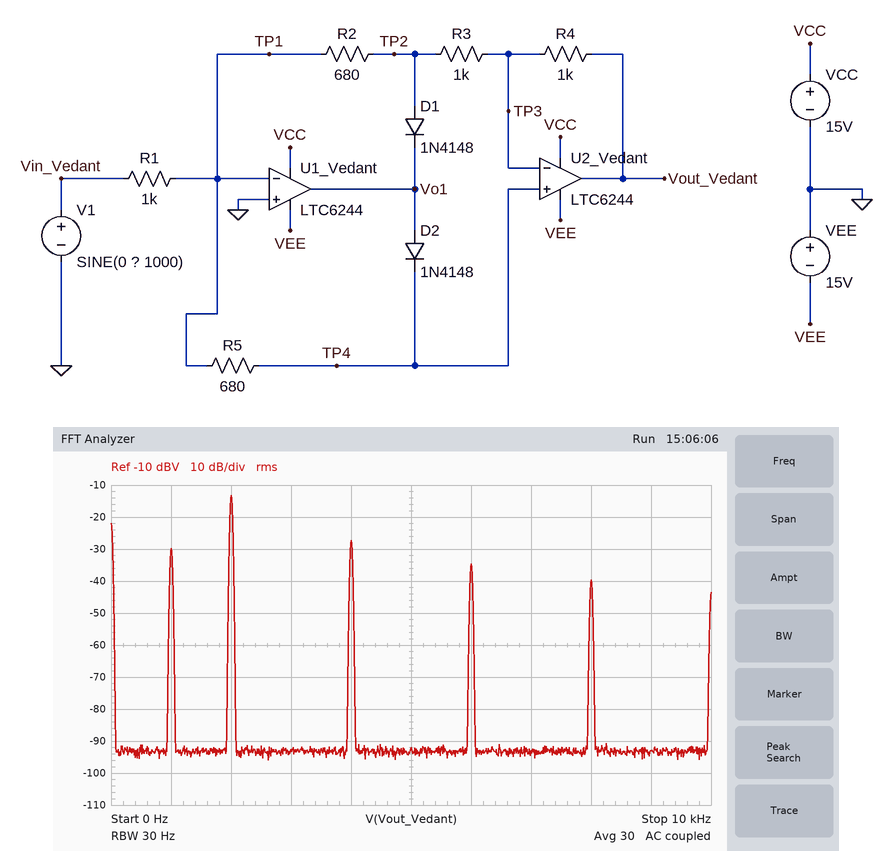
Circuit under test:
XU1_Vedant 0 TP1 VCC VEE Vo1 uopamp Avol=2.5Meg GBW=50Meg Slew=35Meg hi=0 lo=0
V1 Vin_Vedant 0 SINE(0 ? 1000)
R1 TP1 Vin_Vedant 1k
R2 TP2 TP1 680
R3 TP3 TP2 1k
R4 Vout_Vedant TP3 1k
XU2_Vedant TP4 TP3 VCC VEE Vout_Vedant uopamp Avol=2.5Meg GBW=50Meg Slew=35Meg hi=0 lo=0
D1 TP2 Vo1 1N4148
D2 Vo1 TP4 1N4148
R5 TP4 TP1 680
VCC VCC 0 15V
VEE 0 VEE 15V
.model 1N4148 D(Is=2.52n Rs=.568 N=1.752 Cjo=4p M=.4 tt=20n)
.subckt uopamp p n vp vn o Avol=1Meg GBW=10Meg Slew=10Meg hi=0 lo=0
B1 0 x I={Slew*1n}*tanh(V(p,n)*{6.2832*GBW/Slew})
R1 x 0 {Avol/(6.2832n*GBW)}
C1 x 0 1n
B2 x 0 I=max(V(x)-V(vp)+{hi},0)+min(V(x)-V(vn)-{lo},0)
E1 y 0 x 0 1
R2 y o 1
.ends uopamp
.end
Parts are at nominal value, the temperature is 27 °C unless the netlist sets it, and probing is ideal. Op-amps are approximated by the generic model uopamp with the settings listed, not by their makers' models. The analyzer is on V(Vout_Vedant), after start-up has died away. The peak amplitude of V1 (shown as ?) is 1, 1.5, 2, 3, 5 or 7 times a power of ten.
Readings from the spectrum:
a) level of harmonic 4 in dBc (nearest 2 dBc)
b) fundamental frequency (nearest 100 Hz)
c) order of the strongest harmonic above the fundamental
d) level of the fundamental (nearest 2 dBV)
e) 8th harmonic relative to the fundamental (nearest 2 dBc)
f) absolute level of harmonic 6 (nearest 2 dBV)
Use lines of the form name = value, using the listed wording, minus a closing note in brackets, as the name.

level of harmonic 4 in dBc = 2 dBc
fundamental frequency = 1.0 kHz
order of the strongest harmonic above the fundamental = 2
level of the fundamental = -30 dBV
8th harmonic relative to the fundamental = -10 dBc
absolute level of harmonic 6 = -34 dBV
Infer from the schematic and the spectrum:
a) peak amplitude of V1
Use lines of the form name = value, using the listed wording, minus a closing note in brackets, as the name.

peak amplitude of V1 = 1 V
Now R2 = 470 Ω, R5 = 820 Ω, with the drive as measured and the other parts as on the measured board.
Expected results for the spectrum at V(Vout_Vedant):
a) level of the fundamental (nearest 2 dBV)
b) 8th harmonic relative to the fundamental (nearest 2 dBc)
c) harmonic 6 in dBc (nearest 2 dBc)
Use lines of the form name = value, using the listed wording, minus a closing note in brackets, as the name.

level of the fundamental = -16 dBV
8th harmonic relative to the fundamental = -24 dBc
harmonic 6 in dBc = -18 dBc
